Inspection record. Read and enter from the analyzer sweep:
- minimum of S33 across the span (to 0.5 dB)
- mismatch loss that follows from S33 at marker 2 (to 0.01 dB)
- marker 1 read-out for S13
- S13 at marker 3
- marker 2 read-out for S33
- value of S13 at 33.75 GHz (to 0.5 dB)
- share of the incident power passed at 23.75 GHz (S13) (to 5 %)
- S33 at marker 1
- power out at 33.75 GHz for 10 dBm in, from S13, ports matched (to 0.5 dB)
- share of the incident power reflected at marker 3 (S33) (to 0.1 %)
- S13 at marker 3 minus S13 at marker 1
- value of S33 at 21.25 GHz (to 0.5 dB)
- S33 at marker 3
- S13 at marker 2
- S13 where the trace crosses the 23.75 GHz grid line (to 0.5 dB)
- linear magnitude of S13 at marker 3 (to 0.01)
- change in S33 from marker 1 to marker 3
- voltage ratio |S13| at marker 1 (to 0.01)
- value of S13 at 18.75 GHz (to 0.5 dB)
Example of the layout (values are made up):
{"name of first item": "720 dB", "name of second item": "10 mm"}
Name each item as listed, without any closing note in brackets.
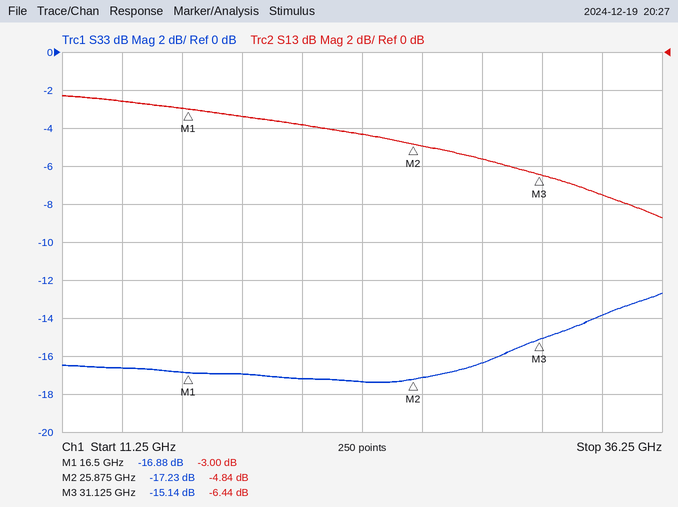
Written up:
{"minimum of S33 across the span": "-17.5 dB", "mismatch loss that follows from S33 at marker 2": "0.08 dB", "marker 1 read-out for S13": "-3.00 dB", "S13 at marker 3": "-6.44 dB", "marker 2 read-out for S33": "-17.23 dB", "value of S13 at 33.75 GHz": "-7.5 dB", "share of the incident power passed at 23.75 GHz (S13)": "35 %", "S33 at marker 1": "-16.88 dB", "power out at 33.75 GHz for 10 dBm in, from S13, ports matched": "2.5 dBm", "share of the incident power reflected at marker 3 (S33)": "3.1 %", "S13 at marker 3 minus S13 at marker 1": "-3.44 dB", "value of S33 at 21.25 GHz": "-17.0 dB", "S33 at marker 3": "-15.14 dB", "S13 at marker 2": "-4.84 dB", "S13 where the trace crosses the 23.75 GHz grid line": "-4.5 dB", "linear magnitude of S13 at marker 3": "0.48", "change in S33 from marker 1 to marker 3": "1.74 dB", "voltage ratio |S13| at marker 1": "0.71", "value of S13 at 18.75 GHz": "-3.5 dB"}
